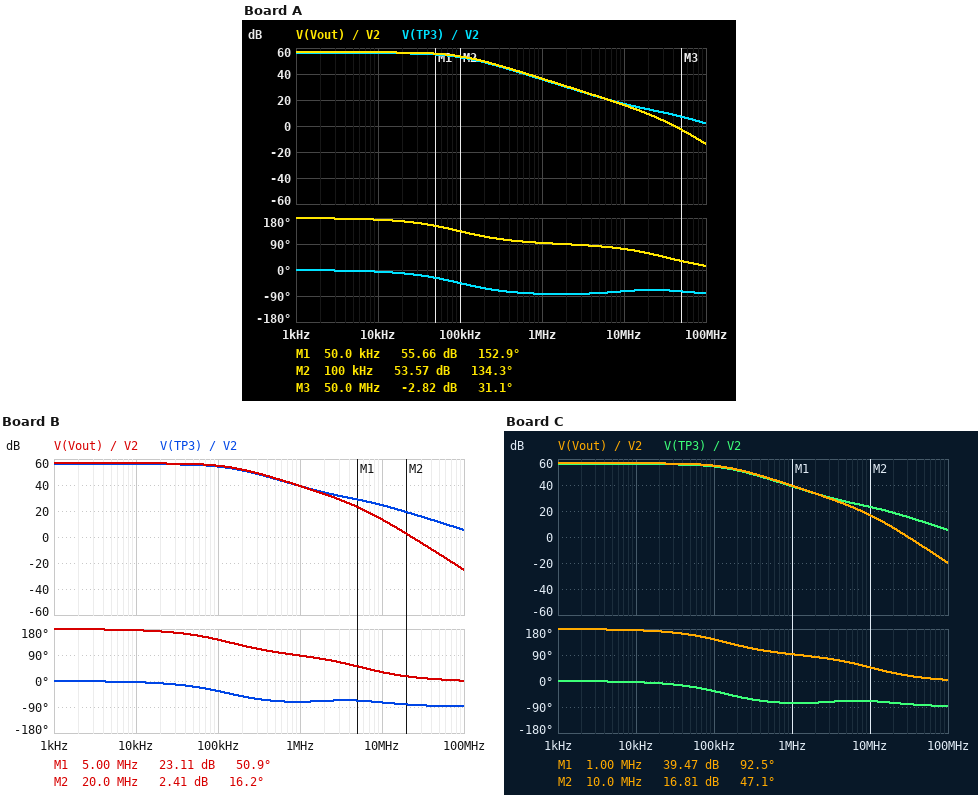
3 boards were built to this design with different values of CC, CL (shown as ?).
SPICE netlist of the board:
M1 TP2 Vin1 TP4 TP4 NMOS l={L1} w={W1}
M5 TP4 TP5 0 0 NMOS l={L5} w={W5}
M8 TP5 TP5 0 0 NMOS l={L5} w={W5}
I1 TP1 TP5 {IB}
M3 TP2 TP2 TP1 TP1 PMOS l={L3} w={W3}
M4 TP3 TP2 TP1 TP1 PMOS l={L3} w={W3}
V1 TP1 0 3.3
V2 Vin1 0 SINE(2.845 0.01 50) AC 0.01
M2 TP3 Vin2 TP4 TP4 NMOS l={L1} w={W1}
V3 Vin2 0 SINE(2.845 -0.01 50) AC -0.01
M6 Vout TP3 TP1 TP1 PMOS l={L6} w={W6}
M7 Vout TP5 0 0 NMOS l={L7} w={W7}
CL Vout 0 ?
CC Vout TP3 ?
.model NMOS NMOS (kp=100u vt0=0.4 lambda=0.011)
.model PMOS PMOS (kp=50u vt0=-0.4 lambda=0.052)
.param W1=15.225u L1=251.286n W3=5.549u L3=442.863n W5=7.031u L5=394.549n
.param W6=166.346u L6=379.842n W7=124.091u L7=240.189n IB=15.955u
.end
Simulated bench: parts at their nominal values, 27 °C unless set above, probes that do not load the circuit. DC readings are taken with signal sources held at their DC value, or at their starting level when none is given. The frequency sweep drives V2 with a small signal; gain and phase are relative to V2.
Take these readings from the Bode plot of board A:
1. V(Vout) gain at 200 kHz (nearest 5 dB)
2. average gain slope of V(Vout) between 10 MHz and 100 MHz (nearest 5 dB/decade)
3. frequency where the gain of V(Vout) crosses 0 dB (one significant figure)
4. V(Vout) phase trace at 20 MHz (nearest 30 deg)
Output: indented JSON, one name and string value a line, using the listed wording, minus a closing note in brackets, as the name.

{
  "V(Vout) gain at 200 kHz": "50 dB",
  "average gain slope of V(Vout) between 10 MHz and 100 MHz": "-30 dB/decade",
  "frequency where the gain of V(Vout) crosses 0 dB": "40 MHz",
  "V(Vout) phase trace at 20 MHz": "60 deg"
}
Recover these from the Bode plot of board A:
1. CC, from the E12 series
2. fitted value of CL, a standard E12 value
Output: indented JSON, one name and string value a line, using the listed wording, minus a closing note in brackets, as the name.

{
  "CC, from the E12 series": "390 fF",
  "fitted value of CL, a standard E12 value": "39 pF"
}
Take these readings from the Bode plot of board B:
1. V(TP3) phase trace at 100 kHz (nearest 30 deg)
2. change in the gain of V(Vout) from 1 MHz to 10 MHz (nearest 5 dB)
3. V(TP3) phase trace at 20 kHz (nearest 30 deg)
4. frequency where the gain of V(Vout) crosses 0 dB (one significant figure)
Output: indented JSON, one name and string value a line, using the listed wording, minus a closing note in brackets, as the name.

{
  "V(TP3) phase trace at 100 kHz": "-30 deg",
  "change in the gain of V(Vout) from 1 MHz to 10 MHz": "-25 dB",
  "V(TP3) phase trace at 20 kHz": "0 deg",
  "frequency where the gain of V(Vout) crosses 0 dB": "20 MHz"
}
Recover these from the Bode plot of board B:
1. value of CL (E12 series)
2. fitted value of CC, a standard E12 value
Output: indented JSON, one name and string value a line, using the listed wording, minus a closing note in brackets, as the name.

{
  "value of CL": "220 pF",
  "fitted value of CC, a standard E12 value": "270 fF"
}
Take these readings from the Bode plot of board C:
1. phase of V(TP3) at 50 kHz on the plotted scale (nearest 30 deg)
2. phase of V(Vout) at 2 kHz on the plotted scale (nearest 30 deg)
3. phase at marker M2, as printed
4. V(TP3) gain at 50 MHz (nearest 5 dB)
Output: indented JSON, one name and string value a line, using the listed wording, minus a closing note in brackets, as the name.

{
  "phase of V(TP3) at 50 kHz on the plotted scale": "-30 deg",
  "phase of V(Vout) at 2 kHz on the plotted scale": "180 deg",
  "phase at marker M2, as printed": "47.1 deg",
  "V(TP3) gain at 50 MHz": "10 dB"
}
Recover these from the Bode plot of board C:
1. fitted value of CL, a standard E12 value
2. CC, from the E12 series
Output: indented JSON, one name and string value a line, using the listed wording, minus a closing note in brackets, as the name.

{
  "fitted value of CL, a standard E12 value": "120 pF",
  "CC, from the E12 series": "270 fF"
}
